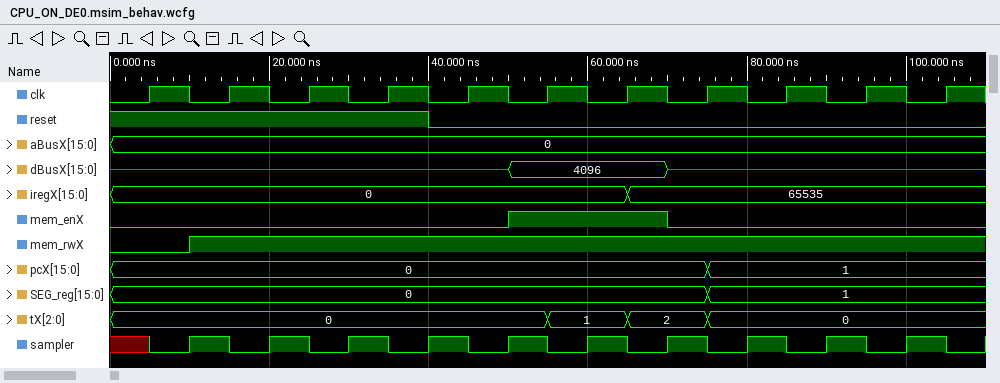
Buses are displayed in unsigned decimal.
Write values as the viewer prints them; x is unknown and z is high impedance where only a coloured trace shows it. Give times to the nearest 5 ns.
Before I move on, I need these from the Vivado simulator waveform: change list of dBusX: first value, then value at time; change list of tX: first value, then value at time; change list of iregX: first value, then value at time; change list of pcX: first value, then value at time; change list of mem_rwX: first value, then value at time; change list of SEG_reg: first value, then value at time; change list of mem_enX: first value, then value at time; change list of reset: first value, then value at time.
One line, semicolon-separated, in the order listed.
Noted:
z, 4096 at 50 ns, z at 70 ns; 0, 1 at 55 ns, 2 at 65 ns, 0 at 75 ns; 0, 65535 at 65 ns; 0, 1 at 75 ns; 0, 1 at 10 ns; 0, 1 at 75 ns; 0, 1 at 50 ns, 0 at 70 ns; 1, 0 at 40 ns
